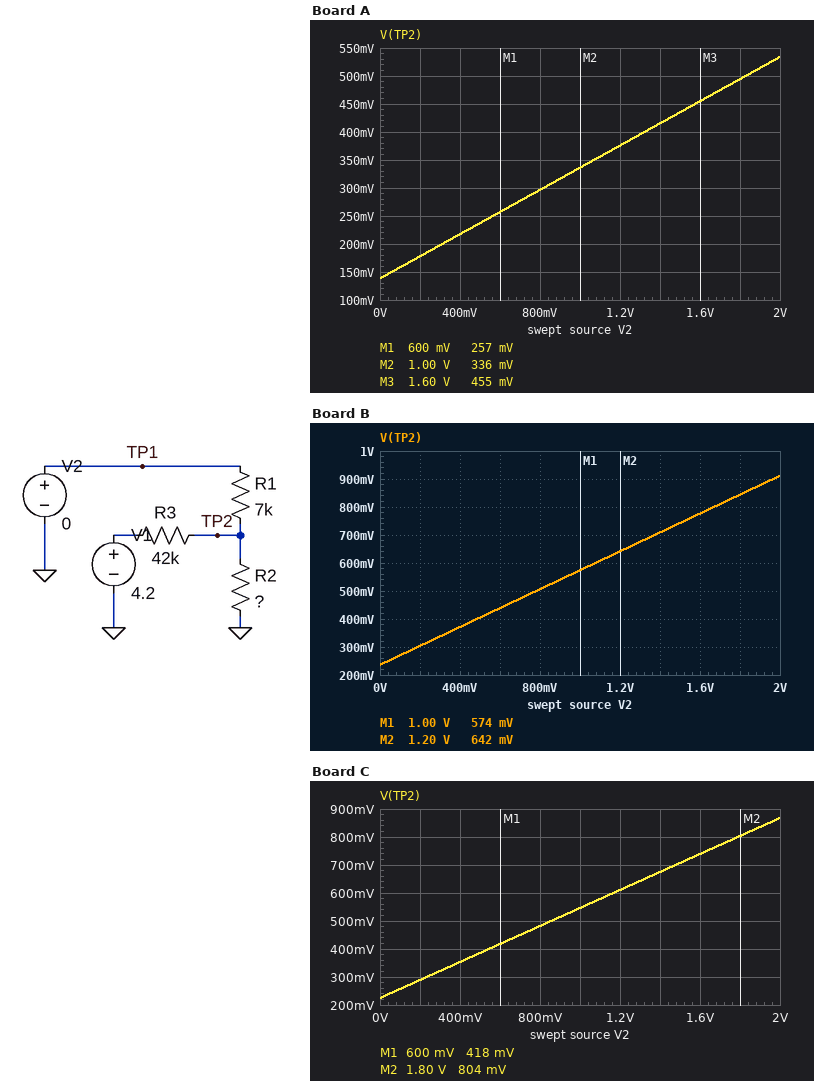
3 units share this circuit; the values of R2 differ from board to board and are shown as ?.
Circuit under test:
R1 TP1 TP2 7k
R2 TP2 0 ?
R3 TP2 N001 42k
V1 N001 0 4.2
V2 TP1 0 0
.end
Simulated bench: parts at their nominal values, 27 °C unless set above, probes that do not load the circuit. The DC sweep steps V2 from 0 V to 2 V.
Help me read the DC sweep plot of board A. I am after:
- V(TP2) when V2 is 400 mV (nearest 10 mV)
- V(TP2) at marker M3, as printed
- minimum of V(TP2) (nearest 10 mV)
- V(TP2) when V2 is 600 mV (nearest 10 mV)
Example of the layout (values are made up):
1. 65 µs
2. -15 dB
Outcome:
1. 220 mV
2. 455 mV
3. 140 mV
4. 260 mV
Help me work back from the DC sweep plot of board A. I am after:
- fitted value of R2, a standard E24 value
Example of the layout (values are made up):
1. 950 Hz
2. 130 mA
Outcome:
1. 1.8 kΩ
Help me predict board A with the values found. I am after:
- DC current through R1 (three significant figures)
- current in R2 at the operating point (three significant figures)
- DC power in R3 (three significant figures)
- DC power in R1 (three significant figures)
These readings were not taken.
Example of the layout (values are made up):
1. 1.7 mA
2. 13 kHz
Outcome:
1. 19.8 µA
2. 76.9 µA
3. 393 µW
4. 2.74 µW
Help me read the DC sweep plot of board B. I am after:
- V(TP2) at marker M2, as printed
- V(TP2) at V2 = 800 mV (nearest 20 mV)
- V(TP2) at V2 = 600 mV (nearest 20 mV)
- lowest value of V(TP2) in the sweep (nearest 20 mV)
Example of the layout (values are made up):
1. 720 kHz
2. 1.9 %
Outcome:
1. 642 mV
2. 500 mV
3. 440 mV
4. 240 mV
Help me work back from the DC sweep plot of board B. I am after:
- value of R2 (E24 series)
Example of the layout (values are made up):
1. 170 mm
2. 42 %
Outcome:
1. 3.9 kΩ
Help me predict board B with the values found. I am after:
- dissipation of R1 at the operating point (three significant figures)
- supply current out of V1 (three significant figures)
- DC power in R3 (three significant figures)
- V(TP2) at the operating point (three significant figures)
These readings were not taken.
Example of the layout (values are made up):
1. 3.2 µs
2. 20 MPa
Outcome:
1. 7.98 µW
2. 94.4 µA
3. 374 µW
4. 236 mV
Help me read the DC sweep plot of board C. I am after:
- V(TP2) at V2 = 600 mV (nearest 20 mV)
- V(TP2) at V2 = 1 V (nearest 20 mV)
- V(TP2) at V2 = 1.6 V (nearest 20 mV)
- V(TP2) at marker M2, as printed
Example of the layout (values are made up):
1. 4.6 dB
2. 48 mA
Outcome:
1. 420 mV
2. 540 mV
3. 740 mV
4. 804 mV
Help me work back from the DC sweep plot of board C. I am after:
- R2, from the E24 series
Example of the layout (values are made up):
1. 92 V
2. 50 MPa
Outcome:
1. 3.6 kΩ
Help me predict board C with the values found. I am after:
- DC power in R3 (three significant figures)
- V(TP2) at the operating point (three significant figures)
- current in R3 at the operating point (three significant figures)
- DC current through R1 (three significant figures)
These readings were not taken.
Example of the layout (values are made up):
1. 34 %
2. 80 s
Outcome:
1. 376 µW
2. 225 mV
3. 94.6 µA
4. 32.1 µA
